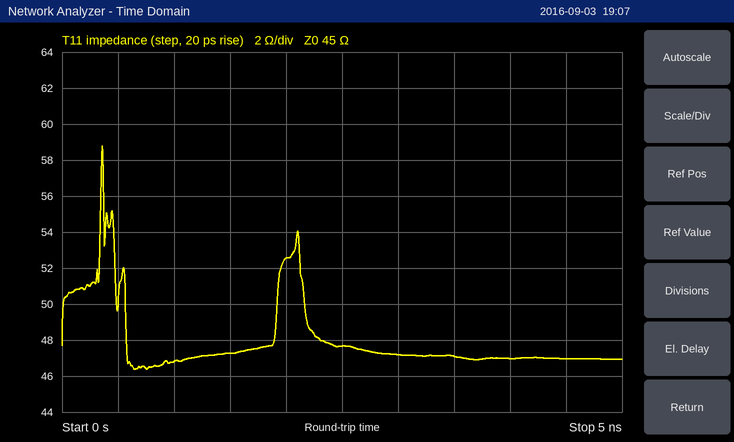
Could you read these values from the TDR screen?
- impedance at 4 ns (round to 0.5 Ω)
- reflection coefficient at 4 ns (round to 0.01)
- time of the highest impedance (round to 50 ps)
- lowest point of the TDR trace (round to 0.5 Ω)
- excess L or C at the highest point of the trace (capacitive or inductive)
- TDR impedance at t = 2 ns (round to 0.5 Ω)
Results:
47.0 Ω
+0.02
350 ps
46.5 Ω
inductive
52.5 Ω
